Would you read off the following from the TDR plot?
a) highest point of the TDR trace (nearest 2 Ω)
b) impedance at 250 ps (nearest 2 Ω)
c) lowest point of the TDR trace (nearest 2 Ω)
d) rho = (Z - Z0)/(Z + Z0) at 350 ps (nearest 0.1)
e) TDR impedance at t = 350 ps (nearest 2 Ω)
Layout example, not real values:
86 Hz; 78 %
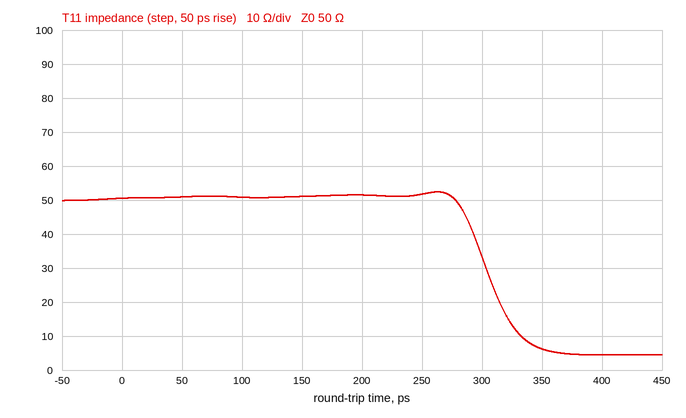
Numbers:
52 Ω; 52 Ω; 4 Ω; -0.8; 6 Ω
